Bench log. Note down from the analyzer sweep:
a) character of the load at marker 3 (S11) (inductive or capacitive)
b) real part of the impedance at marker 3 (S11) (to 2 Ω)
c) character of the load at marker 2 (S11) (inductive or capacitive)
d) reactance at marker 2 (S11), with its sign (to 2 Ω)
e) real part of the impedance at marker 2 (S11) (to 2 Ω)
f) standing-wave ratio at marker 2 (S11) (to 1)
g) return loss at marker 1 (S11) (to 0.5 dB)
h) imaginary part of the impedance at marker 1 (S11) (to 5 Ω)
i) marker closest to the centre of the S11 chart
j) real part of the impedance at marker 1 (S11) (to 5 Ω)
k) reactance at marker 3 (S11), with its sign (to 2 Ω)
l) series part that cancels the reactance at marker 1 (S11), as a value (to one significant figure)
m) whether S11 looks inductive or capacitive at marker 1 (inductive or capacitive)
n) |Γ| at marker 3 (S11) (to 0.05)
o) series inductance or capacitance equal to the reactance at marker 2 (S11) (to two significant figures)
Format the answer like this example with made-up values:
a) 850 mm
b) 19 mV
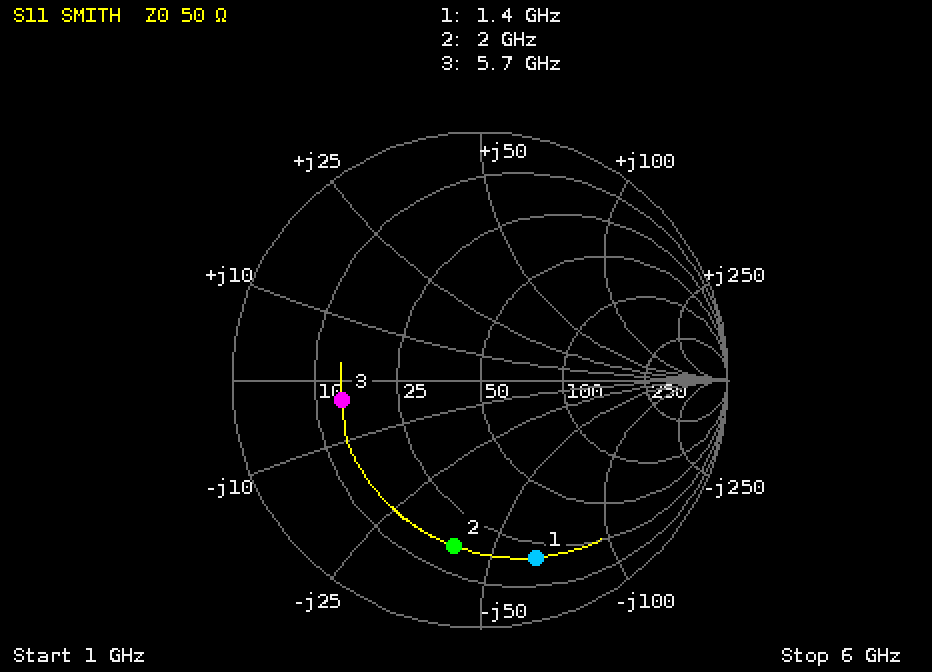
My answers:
a) capacitive
b) 14 Ω
c) capacitive
d) -40 Ω
e) 16 Ω
f) 5
g) 2.5 dB
h) -65 Ω
i) marker 3
j) 20 Ω
k) -4 Ω
l) 7 nH
m) capacitive
n) 0.55
o) 2.0 pF
